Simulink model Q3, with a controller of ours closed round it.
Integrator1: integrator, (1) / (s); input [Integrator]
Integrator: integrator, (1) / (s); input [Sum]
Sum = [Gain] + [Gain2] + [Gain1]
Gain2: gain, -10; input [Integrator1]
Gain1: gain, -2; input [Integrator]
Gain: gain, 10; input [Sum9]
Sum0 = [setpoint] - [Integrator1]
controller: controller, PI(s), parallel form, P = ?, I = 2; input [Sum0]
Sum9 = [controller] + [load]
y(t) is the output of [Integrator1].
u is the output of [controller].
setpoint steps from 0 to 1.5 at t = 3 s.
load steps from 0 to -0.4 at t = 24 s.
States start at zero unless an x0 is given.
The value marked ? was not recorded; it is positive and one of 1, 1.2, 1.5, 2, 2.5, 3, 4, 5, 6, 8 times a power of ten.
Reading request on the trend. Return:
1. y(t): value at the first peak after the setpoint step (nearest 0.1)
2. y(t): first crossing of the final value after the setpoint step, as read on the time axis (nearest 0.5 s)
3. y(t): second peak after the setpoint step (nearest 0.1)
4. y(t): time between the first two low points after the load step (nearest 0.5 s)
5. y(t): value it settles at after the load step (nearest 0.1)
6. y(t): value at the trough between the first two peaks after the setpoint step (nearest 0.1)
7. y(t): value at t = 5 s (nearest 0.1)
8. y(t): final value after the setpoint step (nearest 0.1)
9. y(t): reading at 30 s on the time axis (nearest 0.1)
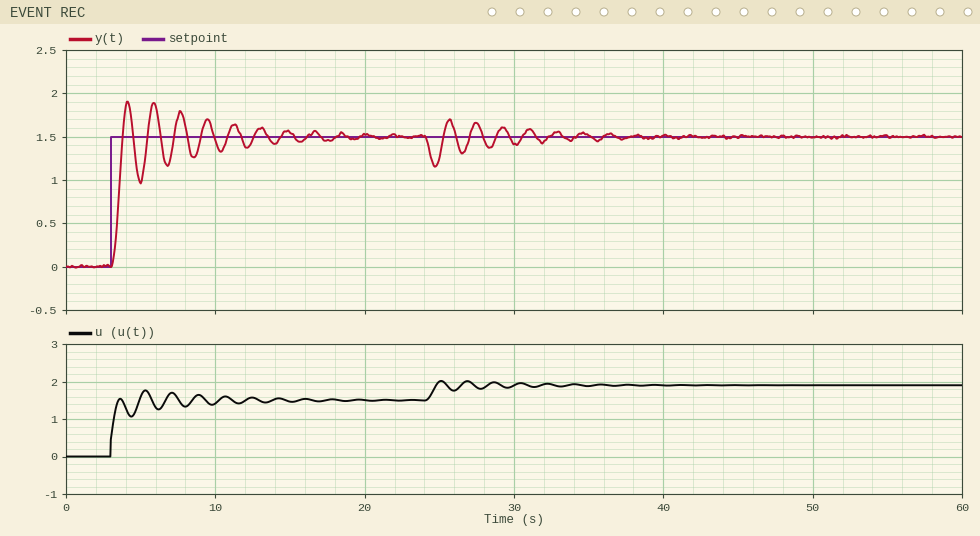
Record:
1.9
4.0 s
1.9
2.0 s
1.5
1.0
1.0
1.5
1.4
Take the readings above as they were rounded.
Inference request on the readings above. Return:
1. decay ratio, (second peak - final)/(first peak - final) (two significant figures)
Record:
1.0
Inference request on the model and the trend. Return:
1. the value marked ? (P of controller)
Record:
0.3
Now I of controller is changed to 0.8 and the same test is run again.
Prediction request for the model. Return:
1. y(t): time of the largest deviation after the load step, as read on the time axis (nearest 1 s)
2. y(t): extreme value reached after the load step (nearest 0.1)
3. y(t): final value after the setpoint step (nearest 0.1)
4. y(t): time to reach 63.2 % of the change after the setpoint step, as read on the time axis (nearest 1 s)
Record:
25 s
1.1
1.5
4 s
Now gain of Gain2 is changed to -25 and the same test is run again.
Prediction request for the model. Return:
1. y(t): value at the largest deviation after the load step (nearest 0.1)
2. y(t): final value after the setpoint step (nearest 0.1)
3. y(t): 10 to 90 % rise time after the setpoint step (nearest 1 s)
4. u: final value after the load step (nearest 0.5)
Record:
1.3
1.5
3 s
4.0
